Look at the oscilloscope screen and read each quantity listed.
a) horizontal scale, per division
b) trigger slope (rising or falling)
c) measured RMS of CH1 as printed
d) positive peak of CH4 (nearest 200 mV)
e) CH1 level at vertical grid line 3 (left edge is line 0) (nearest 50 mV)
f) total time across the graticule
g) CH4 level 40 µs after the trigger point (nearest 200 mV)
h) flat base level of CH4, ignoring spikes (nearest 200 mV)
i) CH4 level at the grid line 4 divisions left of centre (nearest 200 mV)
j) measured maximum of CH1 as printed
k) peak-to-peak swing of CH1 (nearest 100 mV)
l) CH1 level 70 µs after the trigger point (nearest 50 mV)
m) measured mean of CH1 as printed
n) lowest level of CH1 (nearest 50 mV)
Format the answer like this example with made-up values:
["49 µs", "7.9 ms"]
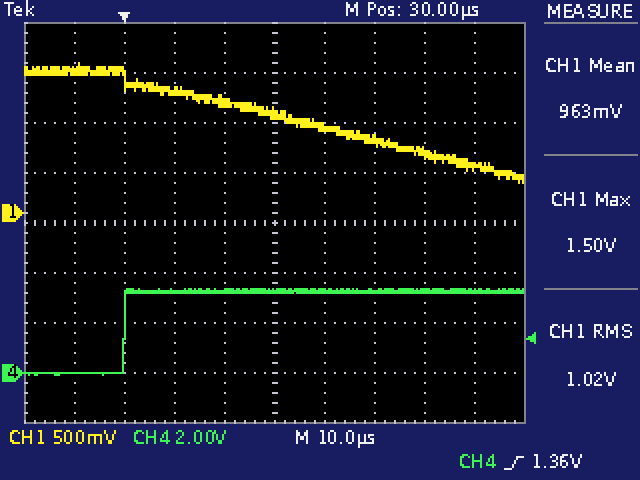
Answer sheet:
["10 µs", "rising", "1.02 V", "3.4 V", "1.20 V", "100 µs", "3.2 V", "0.0 V", "0.0 V", "1.50 V", "1.20 V", "450 mV", "963 mV", "300 mV"]
